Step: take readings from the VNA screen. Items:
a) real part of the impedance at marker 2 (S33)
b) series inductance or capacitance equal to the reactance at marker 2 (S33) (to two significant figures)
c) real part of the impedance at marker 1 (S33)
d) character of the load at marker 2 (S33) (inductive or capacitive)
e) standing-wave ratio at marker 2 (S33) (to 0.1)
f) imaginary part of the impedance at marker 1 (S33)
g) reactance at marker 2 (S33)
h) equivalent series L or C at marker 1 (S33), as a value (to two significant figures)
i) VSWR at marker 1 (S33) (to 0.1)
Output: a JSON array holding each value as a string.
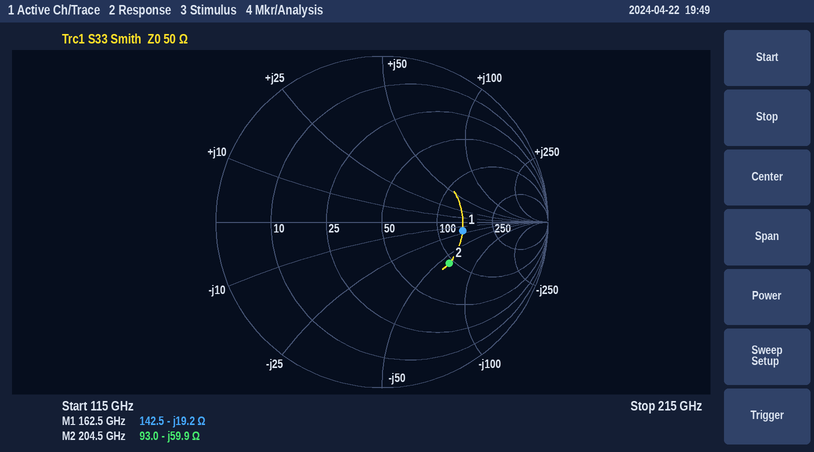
["93.0 Ω", "13 fF", "142.5 Ω", "capacitive", "2.8", "-19.2 Ω", "-59.9 Ω", "51 fF", "2.9"]
